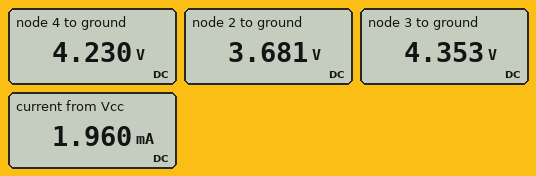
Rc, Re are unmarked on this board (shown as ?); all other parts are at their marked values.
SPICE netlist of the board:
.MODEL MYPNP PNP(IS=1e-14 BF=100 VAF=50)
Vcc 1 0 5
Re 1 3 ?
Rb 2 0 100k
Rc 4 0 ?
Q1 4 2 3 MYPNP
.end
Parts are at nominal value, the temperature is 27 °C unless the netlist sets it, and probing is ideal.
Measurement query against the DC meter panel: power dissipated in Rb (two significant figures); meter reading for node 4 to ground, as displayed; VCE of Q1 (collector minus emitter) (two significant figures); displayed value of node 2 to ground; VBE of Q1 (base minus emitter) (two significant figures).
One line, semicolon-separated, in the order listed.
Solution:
140 µW; 4.230 V; -120 mV; 3.681 V; -670 mV
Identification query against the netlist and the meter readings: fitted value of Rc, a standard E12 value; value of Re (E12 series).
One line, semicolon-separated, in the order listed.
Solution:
2.2 kΩ; 330 Ω
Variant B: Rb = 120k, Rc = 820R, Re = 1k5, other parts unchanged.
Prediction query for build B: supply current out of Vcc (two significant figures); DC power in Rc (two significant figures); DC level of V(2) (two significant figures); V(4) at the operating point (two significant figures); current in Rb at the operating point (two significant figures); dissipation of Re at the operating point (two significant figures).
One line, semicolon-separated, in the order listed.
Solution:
1.6 mA; 2.1 mW; 1.9 V; 1.3 V; 16 µA; 3.9 mW
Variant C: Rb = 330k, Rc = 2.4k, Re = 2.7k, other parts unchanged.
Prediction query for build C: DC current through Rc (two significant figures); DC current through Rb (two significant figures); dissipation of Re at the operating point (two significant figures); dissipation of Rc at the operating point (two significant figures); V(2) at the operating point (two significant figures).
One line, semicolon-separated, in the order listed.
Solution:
730 µA; 7.2 µA; 1.5 mW; 1.3 mW; 2.4 V
